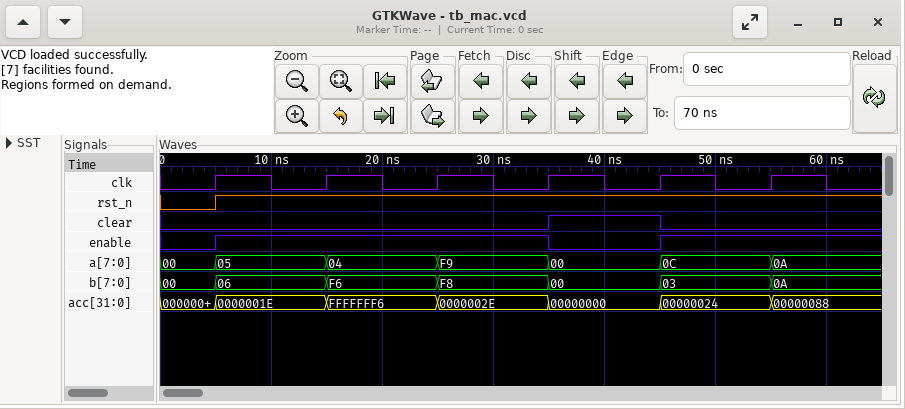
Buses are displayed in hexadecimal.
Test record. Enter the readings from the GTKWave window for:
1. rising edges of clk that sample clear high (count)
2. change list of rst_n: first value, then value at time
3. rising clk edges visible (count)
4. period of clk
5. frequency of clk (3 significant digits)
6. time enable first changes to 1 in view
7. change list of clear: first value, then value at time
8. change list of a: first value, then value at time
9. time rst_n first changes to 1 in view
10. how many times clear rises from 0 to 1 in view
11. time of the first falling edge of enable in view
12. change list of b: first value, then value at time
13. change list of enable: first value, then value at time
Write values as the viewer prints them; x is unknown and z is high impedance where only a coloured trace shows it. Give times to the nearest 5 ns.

1
0, 1 at 5 ns
6
10 ns
100 MHz
5 ns
0, 1 at 35 ns, 0 at 45 ns
00, 05 at 5 ns, 04 at 15 ns, F9 at 25 ns, 00 at 35 ns, 0C at 45 ns, 0A at 55 ns
5 ns
1
35 ns
00, 06 at 5 ns, F6 at 15 ns, F8 at 25 ns, 00 at 35 ns, 03 at 45 ns, 0A at 55 ns
0, 1 at 5 ns, 0 at 35 ns, 1 at 45 ns
